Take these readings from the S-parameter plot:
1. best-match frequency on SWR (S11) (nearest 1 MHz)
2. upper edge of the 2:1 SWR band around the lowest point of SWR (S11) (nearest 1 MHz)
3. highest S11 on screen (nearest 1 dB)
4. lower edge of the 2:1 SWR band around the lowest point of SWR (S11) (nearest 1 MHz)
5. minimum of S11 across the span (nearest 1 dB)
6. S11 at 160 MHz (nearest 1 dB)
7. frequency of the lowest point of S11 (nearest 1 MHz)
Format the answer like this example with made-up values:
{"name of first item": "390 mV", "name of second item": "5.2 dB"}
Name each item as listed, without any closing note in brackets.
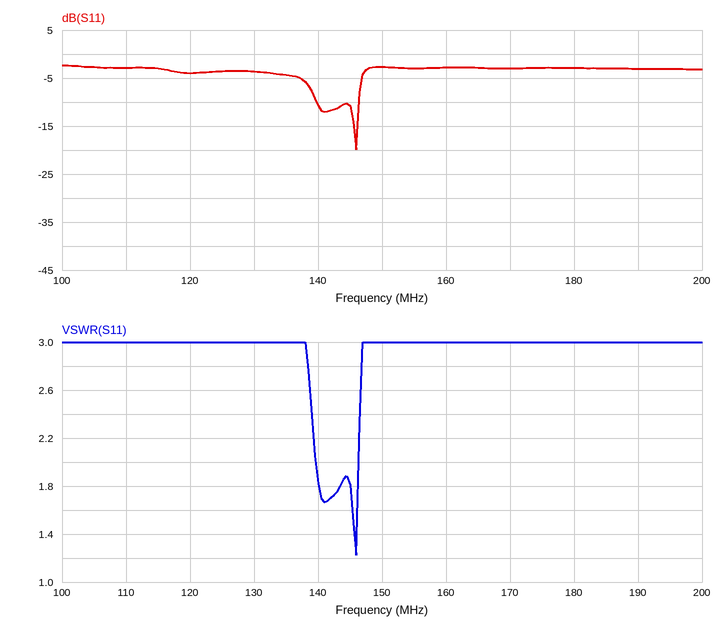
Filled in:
{"best-match frequency on SWR (S11)": "146 MHz", "upper edge of the 2:1 SWR band around the lowest point of SWR (S11)": "146 MHz", "highest S11 on screen": "-2 dB", "lower edge of the 2:1 SWR band around the lowest point of SWR (S11)": "140 MHz", "minimum of S11 across the span": "-20 dB", "S11 at 160 MHz": "-3 dB", "frequency of the lowest point of S11": "146 MHz"}
